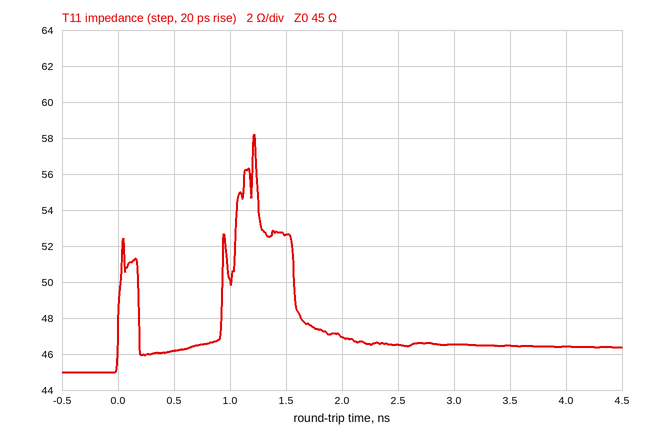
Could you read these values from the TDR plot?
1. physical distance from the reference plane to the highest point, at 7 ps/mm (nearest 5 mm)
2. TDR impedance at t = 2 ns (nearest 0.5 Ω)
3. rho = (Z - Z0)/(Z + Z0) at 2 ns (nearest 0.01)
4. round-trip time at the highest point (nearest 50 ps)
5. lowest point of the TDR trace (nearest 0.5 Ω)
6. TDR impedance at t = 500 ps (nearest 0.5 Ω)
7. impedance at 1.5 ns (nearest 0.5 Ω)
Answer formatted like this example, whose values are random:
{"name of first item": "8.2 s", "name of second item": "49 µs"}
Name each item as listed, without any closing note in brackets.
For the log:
{"physical distance from the reference plane to the highest point, at 7 ps/mm": "85 mm", "TDR impedance at t = 2 ns": "47.0 Ω", "rho = (Z - Z0)/(Z + Z0) at 2 ns": "+0.02", "round-trip time at the highest point": "1.20 ns", "lowest point of the TDR trace": "45.0 Ω", "TDR impedance at t = 500 ps": "46.0 Ω", "impedance at 1.5 ns": "52.5 Ω"}
